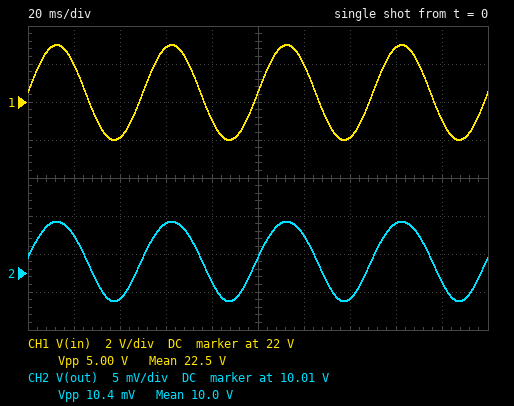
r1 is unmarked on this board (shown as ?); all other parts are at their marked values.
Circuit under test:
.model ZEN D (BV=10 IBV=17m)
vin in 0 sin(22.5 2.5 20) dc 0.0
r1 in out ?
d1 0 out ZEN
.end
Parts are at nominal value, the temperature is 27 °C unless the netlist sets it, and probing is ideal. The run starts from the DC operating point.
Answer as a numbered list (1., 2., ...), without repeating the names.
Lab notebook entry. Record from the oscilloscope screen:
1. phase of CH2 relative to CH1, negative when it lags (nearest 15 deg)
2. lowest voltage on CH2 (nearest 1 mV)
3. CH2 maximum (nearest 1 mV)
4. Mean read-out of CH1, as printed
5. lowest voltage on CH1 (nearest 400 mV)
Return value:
1. 0 deg
2. 10.001 V
3. 10.012 V
4. 22.5 V
5. 20.0 V
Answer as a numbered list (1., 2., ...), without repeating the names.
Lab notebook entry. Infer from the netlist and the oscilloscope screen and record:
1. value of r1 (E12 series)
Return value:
1. 560 Ω
